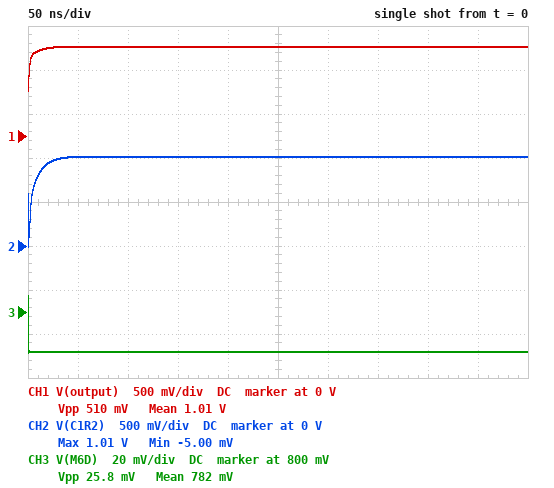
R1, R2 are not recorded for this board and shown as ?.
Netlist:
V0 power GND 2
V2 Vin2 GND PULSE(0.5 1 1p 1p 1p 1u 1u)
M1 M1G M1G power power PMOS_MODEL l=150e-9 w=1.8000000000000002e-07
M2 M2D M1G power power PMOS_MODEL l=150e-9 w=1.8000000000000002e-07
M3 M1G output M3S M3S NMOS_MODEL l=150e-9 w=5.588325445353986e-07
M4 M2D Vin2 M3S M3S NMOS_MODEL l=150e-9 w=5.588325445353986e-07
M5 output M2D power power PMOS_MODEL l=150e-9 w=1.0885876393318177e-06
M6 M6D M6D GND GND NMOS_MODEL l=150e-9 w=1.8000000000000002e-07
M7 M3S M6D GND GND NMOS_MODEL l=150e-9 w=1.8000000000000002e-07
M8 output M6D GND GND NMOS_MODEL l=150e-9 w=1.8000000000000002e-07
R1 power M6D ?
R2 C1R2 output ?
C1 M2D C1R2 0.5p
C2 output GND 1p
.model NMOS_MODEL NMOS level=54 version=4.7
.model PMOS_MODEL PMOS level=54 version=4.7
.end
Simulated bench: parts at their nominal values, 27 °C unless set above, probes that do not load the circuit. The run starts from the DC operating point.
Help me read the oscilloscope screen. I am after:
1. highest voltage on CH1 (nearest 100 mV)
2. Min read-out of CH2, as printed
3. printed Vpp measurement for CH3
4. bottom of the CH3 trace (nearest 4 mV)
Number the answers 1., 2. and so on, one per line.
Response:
1. 1.0 V
2. -5.00 mV
3. 25.8 mV
4. 780 mV
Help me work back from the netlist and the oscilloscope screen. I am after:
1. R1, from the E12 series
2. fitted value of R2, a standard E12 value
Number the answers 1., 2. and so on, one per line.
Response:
1. 33 kΩ
2. 18 kΩ
